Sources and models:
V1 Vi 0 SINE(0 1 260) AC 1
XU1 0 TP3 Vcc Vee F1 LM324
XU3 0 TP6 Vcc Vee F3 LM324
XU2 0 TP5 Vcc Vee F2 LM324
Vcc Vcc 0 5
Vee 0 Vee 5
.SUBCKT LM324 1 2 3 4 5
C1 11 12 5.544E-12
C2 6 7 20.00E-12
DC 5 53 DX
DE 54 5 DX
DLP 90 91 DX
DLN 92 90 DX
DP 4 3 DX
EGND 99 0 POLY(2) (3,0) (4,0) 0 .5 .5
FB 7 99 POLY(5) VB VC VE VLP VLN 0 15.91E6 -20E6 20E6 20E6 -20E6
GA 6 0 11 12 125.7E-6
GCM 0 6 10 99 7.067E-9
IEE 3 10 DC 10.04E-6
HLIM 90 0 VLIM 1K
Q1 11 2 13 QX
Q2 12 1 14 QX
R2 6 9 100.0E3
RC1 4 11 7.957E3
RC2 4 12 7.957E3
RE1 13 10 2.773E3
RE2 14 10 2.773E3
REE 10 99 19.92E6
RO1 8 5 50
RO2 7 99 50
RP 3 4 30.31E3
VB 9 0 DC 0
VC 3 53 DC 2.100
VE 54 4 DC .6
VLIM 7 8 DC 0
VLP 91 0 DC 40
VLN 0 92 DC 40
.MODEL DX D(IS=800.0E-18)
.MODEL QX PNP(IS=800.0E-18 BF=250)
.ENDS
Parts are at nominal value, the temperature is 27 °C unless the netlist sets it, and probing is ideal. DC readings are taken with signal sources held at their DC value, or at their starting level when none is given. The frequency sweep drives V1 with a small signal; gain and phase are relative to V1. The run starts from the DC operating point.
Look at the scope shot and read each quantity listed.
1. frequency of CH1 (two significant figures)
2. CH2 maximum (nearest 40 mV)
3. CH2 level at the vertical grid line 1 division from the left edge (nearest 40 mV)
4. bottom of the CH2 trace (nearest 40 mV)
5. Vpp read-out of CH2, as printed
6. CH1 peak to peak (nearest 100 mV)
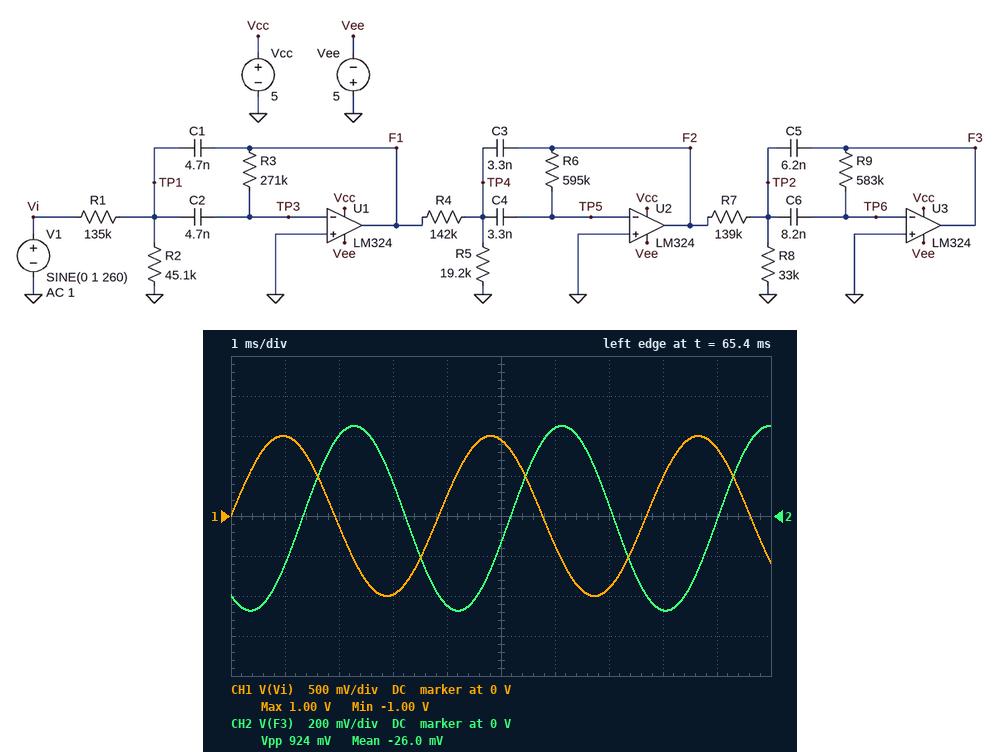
260 Hz
440 mV
-240 mV
-480 mV
924 mV
2.0 V
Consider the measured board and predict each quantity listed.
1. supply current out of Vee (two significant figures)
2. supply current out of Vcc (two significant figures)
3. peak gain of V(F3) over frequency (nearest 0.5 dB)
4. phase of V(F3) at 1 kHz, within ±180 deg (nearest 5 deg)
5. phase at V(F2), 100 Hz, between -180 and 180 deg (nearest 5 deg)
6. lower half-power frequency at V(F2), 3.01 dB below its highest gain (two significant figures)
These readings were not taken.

1.0 mA
1.0 mA
-2.0 dB
-60 deg
165 deg
370 Hz
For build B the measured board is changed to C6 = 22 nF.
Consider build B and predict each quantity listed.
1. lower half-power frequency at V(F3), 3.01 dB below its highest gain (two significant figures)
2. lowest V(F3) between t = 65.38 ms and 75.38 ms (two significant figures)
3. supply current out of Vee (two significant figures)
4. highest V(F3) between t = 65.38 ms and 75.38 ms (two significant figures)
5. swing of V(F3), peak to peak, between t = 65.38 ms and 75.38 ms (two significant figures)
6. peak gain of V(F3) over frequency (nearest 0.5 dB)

320 Hz
-340 mV
1.0 mA
320 mV
660 mV
-3.0 dB
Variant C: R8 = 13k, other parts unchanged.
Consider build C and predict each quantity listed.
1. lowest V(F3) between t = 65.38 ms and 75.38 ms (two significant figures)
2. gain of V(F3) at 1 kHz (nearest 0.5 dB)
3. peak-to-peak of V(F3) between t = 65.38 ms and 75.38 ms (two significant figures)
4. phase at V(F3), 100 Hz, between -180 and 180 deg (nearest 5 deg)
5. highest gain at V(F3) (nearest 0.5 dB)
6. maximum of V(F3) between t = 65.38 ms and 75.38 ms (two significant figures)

-930 mV
-32.5 dB
1.8 V
65 deg
1.5 dB
910 mV
